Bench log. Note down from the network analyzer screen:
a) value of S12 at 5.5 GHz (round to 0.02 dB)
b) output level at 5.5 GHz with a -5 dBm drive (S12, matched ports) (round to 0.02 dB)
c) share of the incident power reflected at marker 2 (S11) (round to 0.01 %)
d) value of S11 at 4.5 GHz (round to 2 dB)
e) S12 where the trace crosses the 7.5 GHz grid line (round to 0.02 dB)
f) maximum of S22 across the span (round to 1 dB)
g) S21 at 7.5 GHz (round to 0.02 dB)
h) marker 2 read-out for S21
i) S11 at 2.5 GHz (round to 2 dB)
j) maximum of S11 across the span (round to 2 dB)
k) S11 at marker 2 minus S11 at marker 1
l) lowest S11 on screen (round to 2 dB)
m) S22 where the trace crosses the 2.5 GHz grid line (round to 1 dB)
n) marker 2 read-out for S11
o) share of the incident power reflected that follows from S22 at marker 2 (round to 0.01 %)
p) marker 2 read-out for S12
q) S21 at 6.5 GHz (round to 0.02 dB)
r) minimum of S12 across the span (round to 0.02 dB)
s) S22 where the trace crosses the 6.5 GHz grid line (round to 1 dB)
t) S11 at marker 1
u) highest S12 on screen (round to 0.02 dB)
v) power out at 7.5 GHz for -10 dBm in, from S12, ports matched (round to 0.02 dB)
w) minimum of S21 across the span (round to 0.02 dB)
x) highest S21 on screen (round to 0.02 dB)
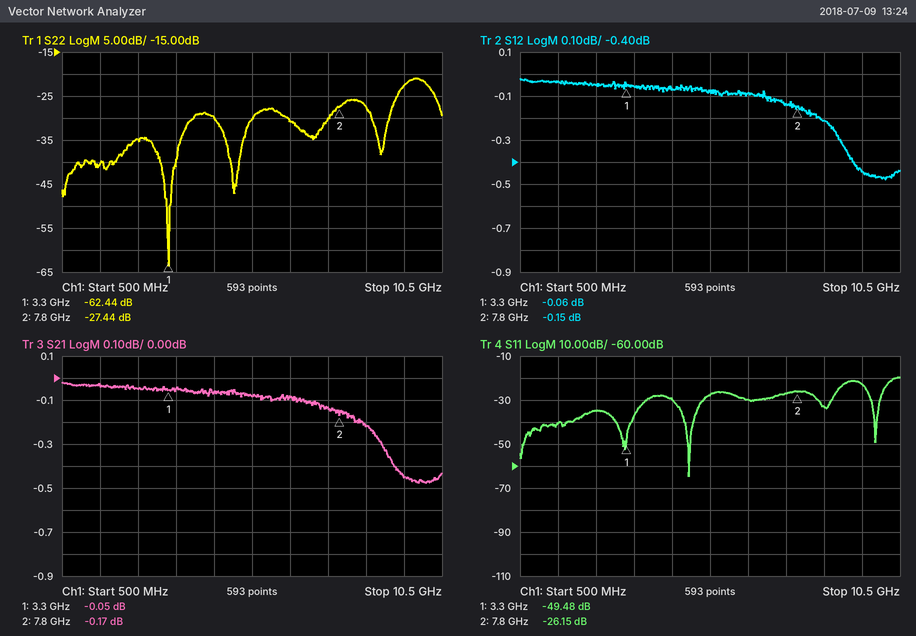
-0.08 dB
-5.08 dBm
0.24 %
-30 dB
-0.14 dB
-21 dB
-0.14 dB
-0.17 dB
-34 dB
-20 dB
23.33 dB
-64 dB
-35 dB
-26.15 dB
0.18 %
-0.15 dB
-0.08 dB
-0.48 dB
-31 dB
-49.48 dB
-0.02 dB
-10.14 dBm
-0.48 dB
-0.02 dB
